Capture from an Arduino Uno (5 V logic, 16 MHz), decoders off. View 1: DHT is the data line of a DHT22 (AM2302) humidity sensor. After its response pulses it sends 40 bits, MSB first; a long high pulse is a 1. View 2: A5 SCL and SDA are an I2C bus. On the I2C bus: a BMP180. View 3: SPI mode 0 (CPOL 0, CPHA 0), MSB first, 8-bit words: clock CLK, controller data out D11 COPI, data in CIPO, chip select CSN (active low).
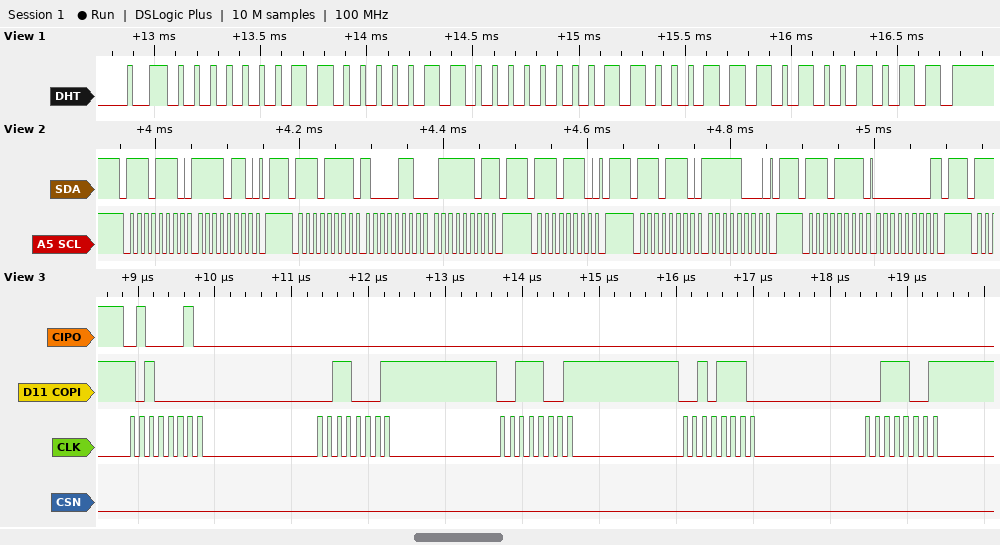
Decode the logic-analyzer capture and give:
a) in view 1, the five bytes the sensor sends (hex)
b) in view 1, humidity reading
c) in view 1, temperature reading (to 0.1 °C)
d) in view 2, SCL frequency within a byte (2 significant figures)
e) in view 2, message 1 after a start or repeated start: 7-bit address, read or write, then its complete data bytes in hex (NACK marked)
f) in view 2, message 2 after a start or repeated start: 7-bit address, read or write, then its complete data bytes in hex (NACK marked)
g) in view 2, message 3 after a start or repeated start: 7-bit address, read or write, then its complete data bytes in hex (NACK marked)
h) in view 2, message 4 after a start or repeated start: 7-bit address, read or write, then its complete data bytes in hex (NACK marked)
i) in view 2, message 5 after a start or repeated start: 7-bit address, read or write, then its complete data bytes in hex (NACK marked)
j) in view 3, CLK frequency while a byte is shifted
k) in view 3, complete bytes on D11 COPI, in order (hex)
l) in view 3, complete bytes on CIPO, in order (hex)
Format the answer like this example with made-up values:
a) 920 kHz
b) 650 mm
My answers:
a) 01 83 00 C7 4B
b) 38.7 %
c) 19.9 °C
d) 100 kHz
e) 0x77 write: F6
f) 0x77 read: 86 7D NACK
g) 0x77 write
h) 0x77 write: F8
i) 0x77 read: 00 NACK
j) 8 MHz
k) A0 31 39 2E 39
l) 42 00 00 00 00
